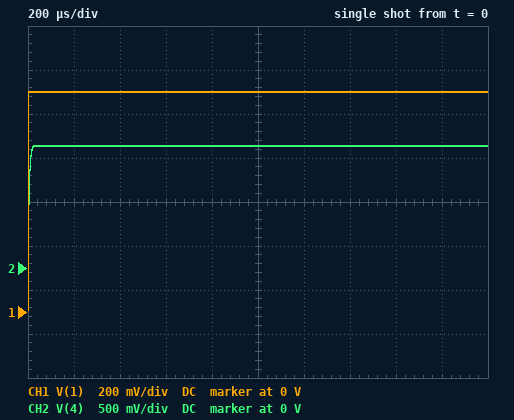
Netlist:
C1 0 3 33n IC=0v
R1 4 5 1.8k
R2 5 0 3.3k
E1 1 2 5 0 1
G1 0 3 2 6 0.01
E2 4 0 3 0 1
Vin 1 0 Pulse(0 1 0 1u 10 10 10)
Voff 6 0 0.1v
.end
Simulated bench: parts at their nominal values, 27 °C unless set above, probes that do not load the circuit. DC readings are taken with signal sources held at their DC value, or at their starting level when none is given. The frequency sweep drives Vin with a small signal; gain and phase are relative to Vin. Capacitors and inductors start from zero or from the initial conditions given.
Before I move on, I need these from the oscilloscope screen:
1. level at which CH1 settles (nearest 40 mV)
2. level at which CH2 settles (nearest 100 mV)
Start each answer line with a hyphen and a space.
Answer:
- 1.00 V
- 1.4 V
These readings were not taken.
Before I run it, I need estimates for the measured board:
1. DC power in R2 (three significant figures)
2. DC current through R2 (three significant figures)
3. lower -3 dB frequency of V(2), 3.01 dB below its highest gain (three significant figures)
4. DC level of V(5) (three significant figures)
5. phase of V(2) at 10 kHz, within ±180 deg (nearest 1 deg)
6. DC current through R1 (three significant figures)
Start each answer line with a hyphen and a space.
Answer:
- 3.03 µW
- 30.3 µA
- 31.2 kHz
- -100 mV
- 72 deg
- 30.3 µA
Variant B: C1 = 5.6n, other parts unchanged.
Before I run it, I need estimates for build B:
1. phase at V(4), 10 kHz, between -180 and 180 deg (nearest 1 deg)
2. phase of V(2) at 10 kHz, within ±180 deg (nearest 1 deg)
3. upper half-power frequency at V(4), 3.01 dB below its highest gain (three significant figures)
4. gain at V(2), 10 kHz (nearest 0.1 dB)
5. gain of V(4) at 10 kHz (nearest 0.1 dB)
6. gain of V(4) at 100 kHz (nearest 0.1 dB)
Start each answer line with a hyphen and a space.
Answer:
- -3 deg
- 87 deg
- 184 kHz
- -25.3 dB
- 3.8 dB
- 2.7 dB
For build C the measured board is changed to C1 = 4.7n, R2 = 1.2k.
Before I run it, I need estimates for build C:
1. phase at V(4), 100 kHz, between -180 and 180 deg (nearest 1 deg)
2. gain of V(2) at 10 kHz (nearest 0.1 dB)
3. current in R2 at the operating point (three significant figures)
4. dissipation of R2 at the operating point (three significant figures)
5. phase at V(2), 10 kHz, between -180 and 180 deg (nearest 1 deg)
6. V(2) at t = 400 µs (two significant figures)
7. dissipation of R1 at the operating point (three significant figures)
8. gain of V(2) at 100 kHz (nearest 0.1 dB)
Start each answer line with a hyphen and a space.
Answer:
- -36 deg
- -22.7 dB
- 83.3 µA
- 8.33 µW
- 86 deg
- 100 mV
- 12.5 µW
- -4.5 dB
